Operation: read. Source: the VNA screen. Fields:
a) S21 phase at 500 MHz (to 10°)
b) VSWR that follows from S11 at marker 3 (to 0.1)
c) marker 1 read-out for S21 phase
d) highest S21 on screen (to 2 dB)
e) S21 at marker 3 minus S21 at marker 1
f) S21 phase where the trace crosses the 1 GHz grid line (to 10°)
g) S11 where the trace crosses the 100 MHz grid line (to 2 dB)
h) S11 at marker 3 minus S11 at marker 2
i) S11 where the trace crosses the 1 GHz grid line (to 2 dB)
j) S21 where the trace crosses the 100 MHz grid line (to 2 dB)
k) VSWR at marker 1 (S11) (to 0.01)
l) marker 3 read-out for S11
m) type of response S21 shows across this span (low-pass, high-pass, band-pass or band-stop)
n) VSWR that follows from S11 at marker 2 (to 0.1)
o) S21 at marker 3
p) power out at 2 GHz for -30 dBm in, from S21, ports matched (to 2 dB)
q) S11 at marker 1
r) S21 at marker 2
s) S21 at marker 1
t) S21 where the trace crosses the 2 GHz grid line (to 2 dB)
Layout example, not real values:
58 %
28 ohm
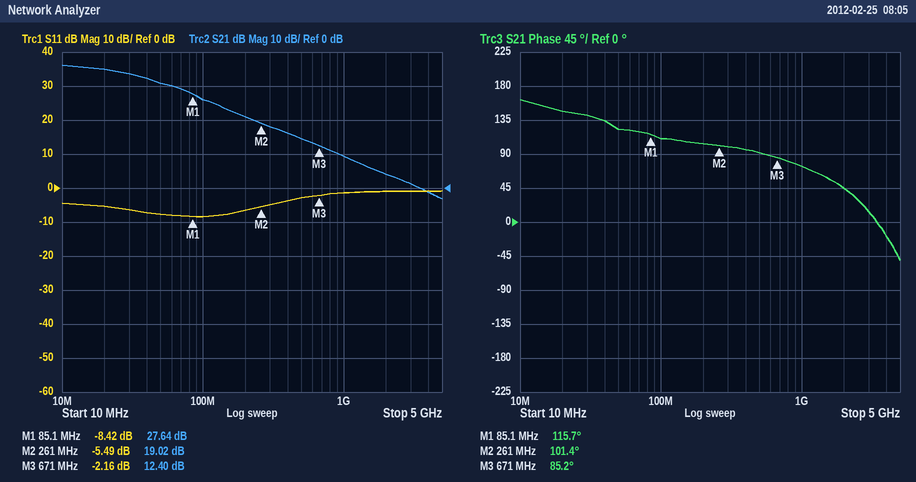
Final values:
90°
8.1
115.7°
36 dB
-15.24 dB
70°
-8 dB
3.33 dB
-2 dB
26 dB
2.22
-2.16 dB
low-pass
3.3
12.40 dB
-26 dBm
-8.42 dB
19.02 dB
27.64 dB
4 dB
